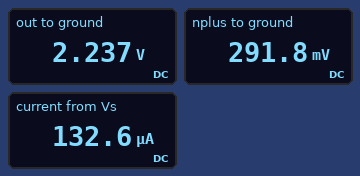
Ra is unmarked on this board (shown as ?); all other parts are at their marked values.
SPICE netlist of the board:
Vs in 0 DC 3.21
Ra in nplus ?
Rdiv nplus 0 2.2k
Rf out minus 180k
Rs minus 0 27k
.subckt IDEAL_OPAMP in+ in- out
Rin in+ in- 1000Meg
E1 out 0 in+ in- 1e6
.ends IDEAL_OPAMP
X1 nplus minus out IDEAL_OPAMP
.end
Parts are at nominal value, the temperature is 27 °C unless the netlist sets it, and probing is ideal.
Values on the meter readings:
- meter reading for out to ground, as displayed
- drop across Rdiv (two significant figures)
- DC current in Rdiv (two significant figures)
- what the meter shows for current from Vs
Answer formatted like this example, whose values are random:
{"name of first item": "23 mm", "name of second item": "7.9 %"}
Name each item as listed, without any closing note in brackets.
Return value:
{"meter reading for out to ground, as displayed": "2.237 V", "drop across Rdiv": "290 mV", "DC current in Rdiv": "130 µA", "what the meter shows for current from Vs": "132.6 µA"}
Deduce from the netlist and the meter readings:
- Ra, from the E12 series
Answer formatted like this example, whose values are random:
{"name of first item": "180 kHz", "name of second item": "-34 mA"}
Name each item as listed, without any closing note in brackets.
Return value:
{"Ra, from the E12 series": "22 kΩ"}
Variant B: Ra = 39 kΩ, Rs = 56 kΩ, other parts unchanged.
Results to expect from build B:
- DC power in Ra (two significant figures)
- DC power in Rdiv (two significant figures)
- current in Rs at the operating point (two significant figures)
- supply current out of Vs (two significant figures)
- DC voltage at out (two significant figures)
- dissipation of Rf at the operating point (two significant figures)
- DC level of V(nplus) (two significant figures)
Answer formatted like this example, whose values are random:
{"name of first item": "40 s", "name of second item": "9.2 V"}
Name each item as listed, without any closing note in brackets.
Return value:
{"DC power in Ra": "240 µW", "DC power in Rdiv": "13 µW", "current in Rs at the operating point": "3.1 µA", "supply current out of Vs": "78 µA", "DC voltage at out": "720 mV", "dissipation of Rf at the operating point": "1.7 µW", "DC level of V(nplus)": "170 mV"}
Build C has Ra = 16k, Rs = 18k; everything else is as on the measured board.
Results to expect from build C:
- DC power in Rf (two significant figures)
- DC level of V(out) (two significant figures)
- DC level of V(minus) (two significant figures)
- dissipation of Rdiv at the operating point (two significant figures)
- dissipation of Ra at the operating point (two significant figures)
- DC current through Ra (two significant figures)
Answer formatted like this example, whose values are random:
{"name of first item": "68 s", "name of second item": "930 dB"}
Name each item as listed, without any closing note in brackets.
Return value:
{"DC power in Rf": "84 µW", "DC level of V(out)": "4.3 V", "DC level of V(minus)": "390 mV", "dissipation of Rdiv at the operating point": "68 µW", "dissipation of Ra at the operating point": "500 µW", "DC current through Ra": "180 µA"}
